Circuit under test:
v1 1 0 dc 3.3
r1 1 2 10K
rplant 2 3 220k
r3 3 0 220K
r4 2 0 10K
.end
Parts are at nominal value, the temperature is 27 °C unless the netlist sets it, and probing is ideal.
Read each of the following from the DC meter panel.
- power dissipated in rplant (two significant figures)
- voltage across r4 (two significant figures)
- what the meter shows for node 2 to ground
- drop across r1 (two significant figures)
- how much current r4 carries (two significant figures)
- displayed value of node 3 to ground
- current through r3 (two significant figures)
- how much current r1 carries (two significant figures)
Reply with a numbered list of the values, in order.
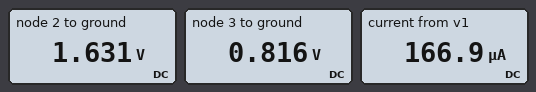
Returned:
1. 3.0 µW
2. 1.6 V
3. 1.631 V
4. 1.7 V
5. 160 µA
6. 0.816 V
7. 3.7 µA
8. 170 µA
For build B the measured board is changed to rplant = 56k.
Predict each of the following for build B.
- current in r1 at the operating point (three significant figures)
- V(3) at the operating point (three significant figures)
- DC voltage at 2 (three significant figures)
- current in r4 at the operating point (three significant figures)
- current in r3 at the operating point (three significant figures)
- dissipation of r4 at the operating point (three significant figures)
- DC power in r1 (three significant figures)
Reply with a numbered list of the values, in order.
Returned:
1. 168 µA
2. 1.29 V
3. 1.62 V
4. 162 µA
5. 5.87 µA
6. 263 µW
7. 282 µW
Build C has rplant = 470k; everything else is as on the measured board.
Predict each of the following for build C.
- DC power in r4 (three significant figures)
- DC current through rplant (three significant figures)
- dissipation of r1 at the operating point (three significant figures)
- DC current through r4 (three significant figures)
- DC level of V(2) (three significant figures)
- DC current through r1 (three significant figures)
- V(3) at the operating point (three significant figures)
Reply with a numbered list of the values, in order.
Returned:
1. 268 µW
2. 2.37 µA
3. 276 µW
4. 164 µA
5. 1.64 V
6. 166 µA
7. 522 mV
